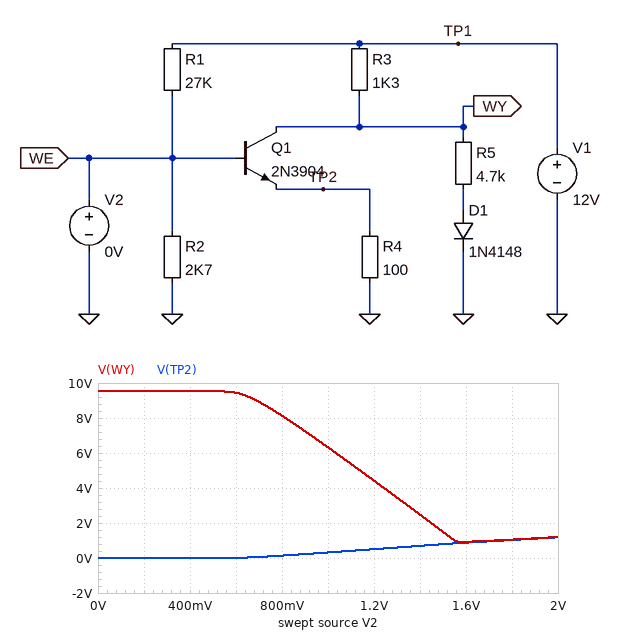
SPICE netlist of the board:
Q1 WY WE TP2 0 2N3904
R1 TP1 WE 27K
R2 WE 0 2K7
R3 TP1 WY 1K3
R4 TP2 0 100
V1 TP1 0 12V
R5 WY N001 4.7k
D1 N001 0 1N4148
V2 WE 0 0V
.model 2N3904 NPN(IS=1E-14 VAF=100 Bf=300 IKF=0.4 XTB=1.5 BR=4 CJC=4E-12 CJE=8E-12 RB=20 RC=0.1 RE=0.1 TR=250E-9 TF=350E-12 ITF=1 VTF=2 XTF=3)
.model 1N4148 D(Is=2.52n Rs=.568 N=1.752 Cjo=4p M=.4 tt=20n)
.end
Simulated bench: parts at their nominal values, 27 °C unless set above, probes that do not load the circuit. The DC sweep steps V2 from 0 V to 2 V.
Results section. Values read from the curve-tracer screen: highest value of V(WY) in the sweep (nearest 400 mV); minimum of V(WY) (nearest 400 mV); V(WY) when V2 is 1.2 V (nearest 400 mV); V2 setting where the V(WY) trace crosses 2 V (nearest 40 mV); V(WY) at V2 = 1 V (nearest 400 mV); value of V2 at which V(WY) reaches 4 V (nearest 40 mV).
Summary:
9.6 V
800 mV
4.4 V
1.44 V
6.4 V
1.24 V
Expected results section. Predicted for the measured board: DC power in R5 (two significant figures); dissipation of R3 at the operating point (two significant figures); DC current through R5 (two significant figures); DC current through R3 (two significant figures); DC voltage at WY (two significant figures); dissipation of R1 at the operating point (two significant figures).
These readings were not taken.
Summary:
17 mW
4.7 mW
1.9 mA
1.9 mA
9.5 V
5.3 mW
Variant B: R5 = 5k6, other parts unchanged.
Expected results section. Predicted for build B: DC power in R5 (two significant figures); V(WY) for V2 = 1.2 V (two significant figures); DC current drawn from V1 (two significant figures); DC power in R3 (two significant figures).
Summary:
15 mW
4.6 V
2.1 mA
3.5 mW
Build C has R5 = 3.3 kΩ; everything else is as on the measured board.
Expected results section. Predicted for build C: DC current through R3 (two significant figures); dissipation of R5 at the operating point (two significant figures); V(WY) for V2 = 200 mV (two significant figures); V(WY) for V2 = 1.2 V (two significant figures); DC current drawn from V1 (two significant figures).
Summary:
2.5 mA
20 mW
8.8 V
4.1 V
2.9 mA
